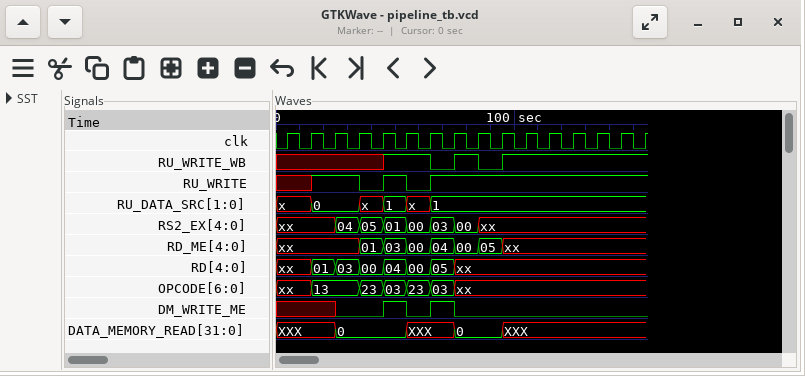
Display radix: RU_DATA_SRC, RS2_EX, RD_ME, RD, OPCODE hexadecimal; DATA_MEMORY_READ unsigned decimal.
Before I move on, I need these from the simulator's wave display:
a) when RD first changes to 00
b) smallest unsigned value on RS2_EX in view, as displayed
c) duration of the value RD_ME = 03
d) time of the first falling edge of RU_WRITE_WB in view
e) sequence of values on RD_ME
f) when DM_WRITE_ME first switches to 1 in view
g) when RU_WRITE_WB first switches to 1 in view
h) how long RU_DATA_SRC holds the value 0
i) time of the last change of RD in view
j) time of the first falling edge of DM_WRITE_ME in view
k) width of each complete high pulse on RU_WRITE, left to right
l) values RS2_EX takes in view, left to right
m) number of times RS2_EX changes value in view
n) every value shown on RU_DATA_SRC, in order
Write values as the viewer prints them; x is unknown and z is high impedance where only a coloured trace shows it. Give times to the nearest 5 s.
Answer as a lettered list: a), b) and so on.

a) 35 s
b) 00
c) 10 s
d) 65 s
e) xx, 01, 03, 00, 04, 00, 05, xx
f) 45 s
g) 45 s
h) 20 s
i) 75 s
j) 55 s
k) 10 s
l) xx, 04, 05, 01, 00, 03, 00, xx
m) 7
n) x, 0, x, 1, x, 1
